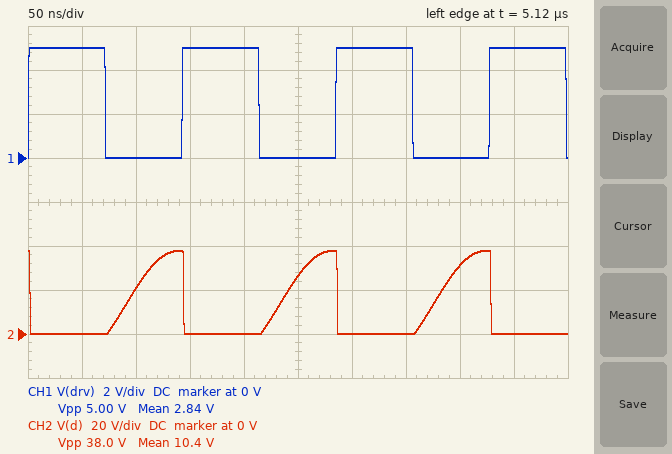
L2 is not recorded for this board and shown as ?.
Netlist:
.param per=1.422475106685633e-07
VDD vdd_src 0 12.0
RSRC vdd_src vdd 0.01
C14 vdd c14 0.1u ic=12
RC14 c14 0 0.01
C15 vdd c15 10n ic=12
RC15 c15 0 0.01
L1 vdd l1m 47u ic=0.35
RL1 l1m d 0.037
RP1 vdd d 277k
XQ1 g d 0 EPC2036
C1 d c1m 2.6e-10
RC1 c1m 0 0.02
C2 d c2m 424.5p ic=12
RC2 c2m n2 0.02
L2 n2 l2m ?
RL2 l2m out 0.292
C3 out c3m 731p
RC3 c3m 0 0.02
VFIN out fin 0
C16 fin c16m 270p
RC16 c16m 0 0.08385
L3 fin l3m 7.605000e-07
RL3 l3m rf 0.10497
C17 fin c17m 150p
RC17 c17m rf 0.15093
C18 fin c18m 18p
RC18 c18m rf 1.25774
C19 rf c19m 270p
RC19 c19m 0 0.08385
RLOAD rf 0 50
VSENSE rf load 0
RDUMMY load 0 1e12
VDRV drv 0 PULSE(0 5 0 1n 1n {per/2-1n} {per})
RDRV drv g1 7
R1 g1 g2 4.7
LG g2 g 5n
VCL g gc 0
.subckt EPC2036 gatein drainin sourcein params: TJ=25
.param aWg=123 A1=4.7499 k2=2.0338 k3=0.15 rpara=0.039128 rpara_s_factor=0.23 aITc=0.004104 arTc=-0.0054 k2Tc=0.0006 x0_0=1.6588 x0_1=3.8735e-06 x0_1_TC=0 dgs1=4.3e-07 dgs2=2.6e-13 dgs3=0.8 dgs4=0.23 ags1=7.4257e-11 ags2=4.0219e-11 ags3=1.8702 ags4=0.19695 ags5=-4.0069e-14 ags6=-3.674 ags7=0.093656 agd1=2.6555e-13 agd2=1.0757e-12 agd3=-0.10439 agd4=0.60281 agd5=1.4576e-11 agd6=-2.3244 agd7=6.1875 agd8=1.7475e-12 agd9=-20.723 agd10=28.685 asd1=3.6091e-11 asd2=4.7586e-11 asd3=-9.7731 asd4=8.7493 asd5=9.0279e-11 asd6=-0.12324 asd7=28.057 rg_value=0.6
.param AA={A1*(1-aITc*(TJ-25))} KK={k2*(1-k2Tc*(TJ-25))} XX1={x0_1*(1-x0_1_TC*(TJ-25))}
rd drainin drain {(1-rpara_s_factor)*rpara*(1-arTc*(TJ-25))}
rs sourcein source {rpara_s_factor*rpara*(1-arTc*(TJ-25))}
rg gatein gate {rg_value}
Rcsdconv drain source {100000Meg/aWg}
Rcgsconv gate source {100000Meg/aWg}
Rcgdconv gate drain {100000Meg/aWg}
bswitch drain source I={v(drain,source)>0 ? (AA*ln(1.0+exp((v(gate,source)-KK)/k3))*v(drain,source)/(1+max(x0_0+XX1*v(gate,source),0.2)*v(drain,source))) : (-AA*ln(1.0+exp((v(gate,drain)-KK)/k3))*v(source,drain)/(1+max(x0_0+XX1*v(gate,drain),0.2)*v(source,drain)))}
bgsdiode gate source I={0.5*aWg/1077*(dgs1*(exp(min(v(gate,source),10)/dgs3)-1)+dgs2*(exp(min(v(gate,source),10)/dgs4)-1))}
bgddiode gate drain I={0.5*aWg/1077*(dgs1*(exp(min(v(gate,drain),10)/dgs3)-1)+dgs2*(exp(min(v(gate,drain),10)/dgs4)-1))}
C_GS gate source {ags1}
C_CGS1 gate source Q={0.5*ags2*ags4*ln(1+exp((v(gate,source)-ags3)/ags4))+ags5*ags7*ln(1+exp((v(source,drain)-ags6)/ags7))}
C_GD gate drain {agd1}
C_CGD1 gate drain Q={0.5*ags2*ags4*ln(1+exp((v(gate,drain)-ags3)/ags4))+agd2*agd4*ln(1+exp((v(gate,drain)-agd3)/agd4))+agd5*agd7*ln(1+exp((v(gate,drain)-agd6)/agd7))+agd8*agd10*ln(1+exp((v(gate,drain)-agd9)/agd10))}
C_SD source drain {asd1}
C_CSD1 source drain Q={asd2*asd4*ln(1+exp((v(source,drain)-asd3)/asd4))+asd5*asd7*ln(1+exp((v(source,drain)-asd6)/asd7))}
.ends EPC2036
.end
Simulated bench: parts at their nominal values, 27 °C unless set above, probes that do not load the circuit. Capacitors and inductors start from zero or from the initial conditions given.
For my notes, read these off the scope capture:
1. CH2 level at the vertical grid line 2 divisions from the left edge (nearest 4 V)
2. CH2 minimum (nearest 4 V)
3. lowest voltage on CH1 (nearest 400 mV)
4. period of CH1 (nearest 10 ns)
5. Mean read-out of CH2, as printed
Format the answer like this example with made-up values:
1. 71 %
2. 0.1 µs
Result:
1. 20 V
2. 0 V
3. 0 V
4. 140 ns
5. 10.4 V
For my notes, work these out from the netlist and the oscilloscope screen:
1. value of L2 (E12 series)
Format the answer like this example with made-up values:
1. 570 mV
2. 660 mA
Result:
1. 4.7 µH
